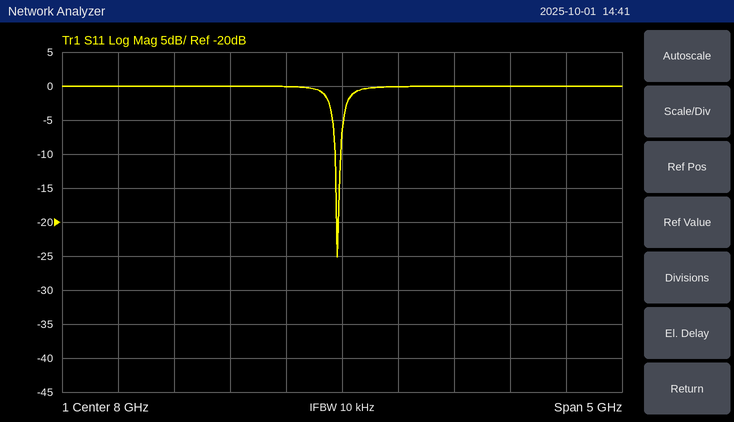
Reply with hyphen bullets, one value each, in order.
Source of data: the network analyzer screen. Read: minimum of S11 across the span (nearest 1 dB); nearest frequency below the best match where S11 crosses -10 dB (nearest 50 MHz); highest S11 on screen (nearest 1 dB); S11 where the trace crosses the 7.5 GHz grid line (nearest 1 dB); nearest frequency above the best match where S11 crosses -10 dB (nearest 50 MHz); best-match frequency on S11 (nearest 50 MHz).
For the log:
- -25 dB
- 7.95 GHz
- 0 dB
- 0 dB
- 8.00 GHz
- 7.95 GHz
